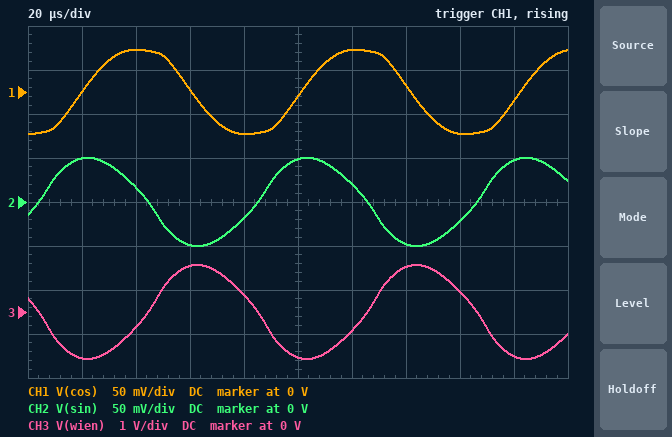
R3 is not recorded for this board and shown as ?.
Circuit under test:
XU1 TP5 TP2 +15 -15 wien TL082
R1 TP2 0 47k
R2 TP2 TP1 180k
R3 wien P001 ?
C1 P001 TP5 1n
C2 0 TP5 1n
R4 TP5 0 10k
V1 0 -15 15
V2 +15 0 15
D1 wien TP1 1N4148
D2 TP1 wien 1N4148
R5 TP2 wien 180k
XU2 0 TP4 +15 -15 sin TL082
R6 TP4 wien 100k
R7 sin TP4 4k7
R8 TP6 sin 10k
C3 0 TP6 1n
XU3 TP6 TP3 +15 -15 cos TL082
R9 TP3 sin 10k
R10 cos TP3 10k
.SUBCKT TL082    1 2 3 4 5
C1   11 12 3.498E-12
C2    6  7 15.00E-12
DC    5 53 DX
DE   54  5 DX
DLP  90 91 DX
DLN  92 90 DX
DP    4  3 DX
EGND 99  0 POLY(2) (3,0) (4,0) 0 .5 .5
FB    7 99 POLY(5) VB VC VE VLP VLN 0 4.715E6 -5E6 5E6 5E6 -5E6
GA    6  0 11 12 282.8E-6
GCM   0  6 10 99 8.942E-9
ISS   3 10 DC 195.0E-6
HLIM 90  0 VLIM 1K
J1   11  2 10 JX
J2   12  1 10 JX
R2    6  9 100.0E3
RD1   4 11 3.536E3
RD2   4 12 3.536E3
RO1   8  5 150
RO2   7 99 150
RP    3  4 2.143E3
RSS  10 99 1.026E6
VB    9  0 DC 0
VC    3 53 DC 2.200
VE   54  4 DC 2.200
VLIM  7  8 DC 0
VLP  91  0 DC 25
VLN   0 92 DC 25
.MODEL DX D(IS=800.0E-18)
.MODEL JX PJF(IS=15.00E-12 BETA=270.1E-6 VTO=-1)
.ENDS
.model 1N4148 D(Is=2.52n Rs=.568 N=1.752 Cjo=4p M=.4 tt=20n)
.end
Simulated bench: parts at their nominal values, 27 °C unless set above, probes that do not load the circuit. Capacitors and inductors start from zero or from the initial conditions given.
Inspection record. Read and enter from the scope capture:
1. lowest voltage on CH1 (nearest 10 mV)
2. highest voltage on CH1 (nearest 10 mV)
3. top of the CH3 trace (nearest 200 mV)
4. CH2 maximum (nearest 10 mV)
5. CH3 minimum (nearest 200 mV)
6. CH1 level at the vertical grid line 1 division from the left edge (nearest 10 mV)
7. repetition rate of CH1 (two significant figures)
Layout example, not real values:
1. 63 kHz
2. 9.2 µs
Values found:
1. -50 mV
2. 50 mV
3. 1.0 V
4. 50 mV
5. -1.0 V
6. 0 V
7. 12 kHz
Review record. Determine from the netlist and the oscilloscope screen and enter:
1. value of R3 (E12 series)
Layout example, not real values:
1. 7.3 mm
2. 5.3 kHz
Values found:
1. 15 kΩ
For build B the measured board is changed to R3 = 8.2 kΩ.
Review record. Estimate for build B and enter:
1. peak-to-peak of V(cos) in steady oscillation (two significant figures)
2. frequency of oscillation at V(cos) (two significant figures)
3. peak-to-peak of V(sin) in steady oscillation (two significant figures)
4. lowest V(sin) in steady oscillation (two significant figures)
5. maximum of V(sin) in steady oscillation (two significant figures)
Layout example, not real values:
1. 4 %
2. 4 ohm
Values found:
1. 1.4 V
2. 17 kHz
3. 1.3 V
4. -630 mV
5. 630 mV
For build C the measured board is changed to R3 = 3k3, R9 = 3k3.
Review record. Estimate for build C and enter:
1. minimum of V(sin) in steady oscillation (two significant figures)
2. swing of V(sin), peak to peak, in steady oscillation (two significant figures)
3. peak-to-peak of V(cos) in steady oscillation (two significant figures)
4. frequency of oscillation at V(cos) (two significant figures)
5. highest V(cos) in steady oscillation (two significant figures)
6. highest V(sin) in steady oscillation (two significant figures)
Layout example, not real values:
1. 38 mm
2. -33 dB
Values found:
1. -630 mV
2. 1.3 V
3. 5.7 V
4. 22 kHz
5. 2.8 V
6. 630 mV
